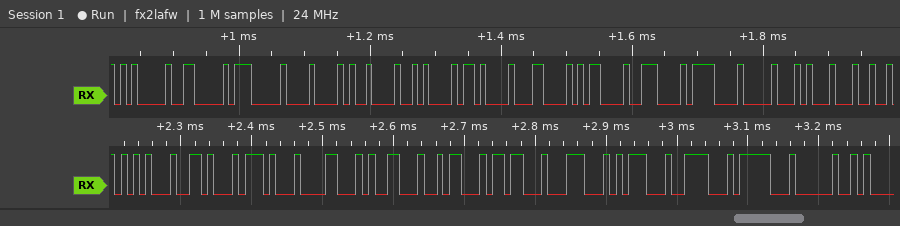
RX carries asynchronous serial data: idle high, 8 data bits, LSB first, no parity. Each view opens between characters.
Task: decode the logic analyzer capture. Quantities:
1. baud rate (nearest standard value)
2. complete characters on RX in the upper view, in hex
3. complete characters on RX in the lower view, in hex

115200 baud
05, 06, 07, 08, 09, 0A, 0B, 0C, 0D, 0E, 0F, 10, 11
15, 16, 17, 18, 19, 1A, 1B, 1C, 1D, 1E, 1F, 20
